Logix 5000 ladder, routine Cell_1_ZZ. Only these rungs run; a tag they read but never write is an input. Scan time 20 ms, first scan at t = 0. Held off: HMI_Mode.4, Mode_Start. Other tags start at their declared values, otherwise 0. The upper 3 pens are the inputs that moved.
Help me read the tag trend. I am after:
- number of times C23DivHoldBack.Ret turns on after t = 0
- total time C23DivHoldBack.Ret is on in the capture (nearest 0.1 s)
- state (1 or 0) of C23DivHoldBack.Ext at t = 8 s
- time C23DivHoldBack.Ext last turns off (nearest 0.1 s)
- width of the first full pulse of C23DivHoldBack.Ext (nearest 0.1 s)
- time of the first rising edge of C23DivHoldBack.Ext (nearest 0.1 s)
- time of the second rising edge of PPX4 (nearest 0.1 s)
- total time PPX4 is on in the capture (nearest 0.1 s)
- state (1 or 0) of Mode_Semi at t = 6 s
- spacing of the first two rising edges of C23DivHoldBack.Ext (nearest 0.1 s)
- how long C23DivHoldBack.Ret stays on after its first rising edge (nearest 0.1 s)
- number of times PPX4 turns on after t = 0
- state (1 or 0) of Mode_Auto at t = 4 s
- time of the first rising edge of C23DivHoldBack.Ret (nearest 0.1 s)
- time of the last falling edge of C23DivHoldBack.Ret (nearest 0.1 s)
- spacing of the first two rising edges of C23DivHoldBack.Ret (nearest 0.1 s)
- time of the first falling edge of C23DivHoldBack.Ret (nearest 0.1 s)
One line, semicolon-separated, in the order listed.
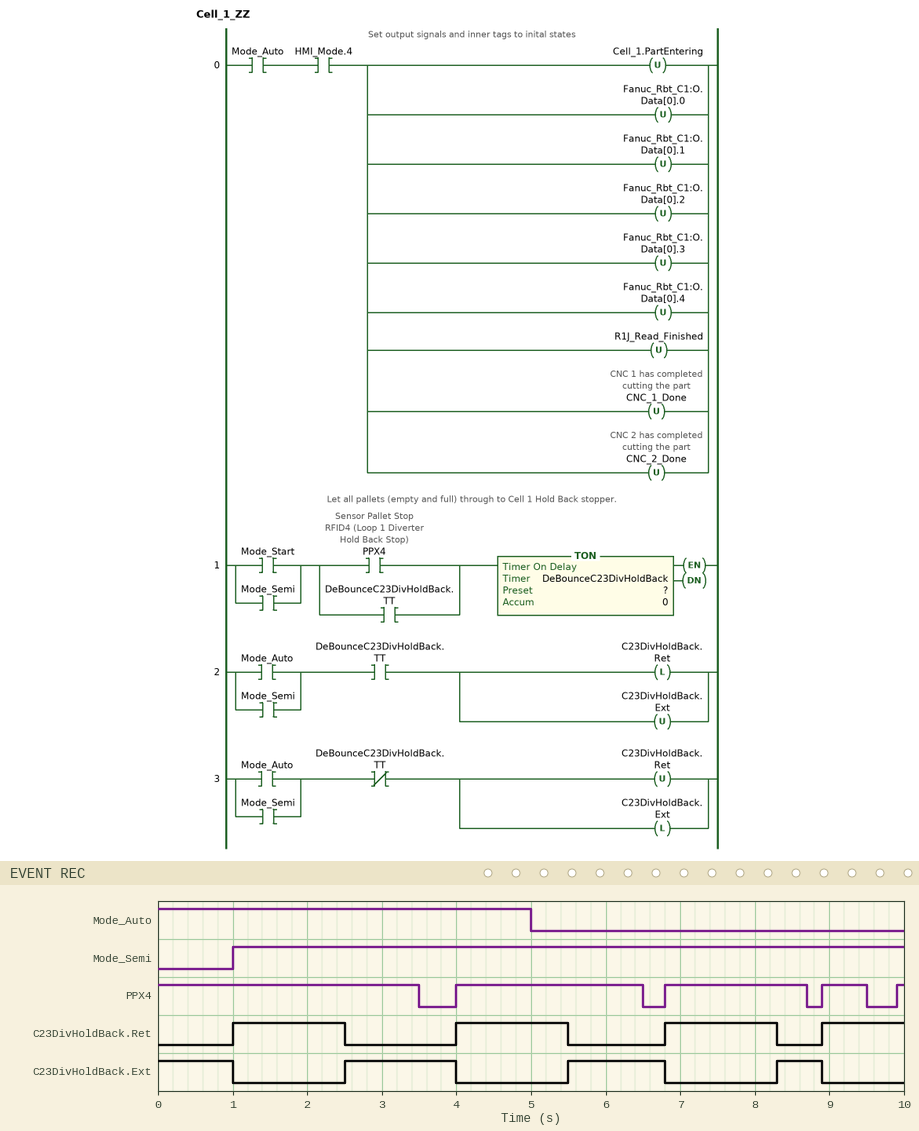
4; 5.6 s; 0; 8.9 s; 1.5 s; 2.5 s; 6.8 s; 8.6 s; 1; 3.0 s; 1.5 s; 4; 1; 1.0 s; 8.3 s; 3.0 s; 2.5 s
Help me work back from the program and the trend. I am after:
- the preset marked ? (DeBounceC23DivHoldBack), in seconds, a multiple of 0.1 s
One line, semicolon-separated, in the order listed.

1.5 s
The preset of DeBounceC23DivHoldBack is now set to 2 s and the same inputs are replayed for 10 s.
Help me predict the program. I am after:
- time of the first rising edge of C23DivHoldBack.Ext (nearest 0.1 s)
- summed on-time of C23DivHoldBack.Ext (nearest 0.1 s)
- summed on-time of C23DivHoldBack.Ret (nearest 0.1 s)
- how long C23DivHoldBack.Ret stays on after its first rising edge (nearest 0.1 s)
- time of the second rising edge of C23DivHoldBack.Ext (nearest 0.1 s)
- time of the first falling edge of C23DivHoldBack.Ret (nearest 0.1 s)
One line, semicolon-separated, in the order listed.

3.0 s; 2.9 s; 7.1 s; 2.0 s; 6.0 s; 3.0 s
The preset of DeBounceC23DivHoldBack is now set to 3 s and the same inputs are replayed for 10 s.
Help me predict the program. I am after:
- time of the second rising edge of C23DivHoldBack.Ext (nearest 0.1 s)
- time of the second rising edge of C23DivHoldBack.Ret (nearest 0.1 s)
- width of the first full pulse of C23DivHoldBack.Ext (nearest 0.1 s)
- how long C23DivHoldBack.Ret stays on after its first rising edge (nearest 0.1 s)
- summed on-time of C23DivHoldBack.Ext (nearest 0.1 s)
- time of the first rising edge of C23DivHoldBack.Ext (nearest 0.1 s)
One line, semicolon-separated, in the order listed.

9.8 s; 6.8 s; 2.8 s; 3.0 s; 3.9 s; 4.0 s
